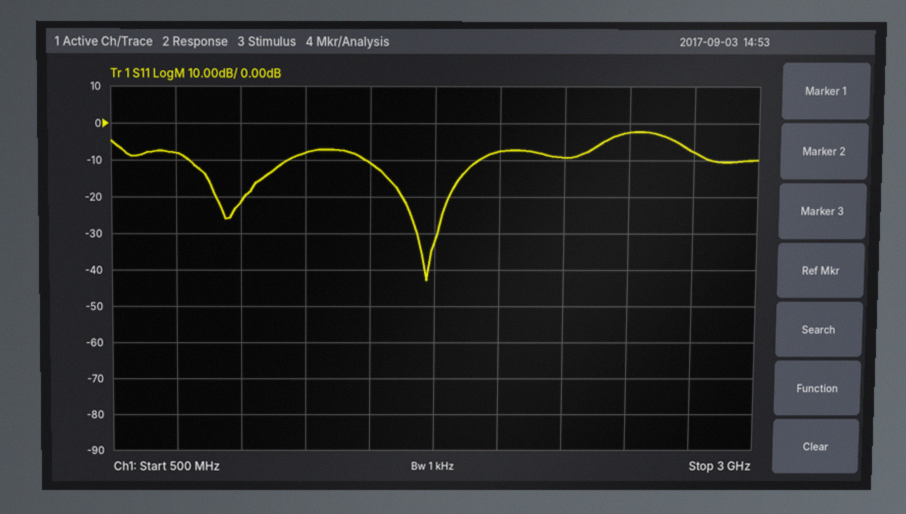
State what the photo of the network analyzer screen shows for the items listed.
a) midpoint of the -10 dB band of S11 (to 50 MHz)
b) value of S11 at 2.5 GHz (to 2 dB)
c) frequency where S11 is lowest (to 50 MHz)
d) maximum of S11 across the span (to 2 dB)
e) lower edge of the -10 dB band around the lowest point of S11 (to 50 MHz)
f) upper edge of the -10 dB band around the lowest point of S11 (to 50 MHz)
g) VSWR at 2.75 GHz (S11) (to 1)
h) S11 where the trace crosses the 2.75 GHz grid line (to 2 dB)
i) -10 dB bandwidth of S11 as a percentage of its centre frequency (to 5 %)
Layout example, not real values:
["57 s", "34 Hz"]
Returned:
["1.70 GHz", "-2 dB", "1.70 GHz", "-2 dB", "1.50 GHz", "1.90 GHz", "2", "-8 dB", "25 %"]
